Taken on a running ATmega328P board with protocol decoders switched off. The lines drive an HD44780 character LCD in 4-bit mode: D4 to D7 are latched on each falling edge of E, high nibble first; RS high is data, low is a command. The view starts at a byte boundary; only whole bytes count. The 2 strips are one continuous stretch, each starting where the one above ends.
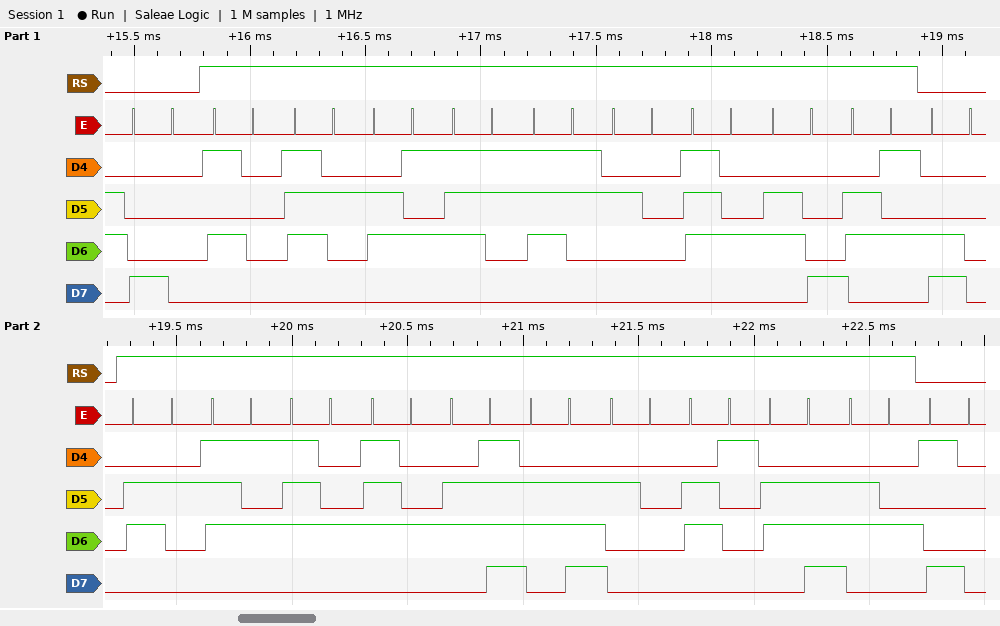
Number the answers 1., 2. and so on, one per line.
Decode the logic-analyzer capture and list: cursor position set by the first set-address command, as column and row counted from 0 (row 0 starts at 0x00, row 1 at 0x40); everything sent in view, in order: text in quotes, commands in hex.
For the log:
1. column 0, row 0
2. 0x80 "Press the" 0xC0 "button and" 0x90
